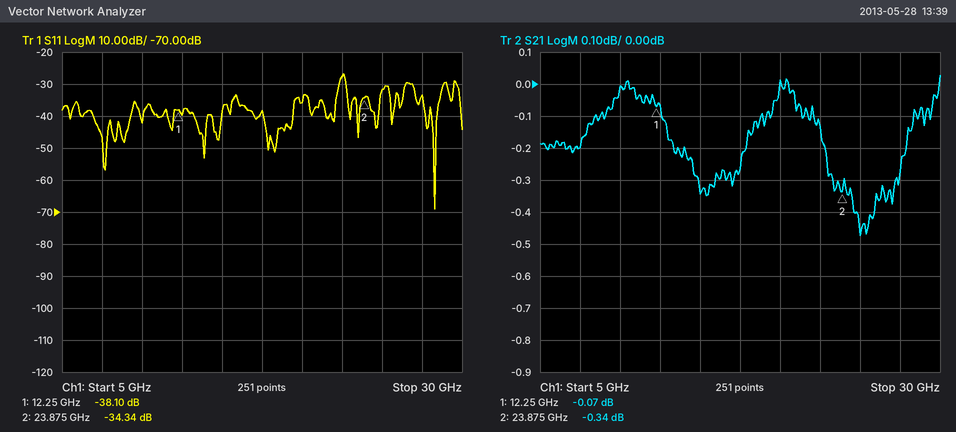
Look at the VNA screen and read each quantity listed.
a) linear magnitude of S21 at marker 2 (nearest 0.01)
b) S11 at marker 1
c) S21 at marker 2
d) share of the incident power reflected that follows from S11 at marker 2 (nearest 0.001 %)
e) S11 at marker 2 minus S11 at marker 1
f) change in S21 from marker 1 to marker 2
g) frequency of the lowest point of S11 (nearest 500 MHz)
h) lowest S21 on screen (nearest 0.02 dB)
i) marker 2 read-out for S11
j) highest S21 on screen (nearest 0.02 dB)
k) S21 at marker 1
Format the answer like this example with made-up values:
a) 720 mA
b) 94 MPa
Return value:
a) 0.96
b) -38.10 dB
c) -0.34 dB
d) 0.037 %
e) 3.76 dB
f) -0.27 dB
g) 28.5 GHz
h) -0.48 dB
i) -34.34 dB
j) 0.02 dB
k) -0.07 dB
